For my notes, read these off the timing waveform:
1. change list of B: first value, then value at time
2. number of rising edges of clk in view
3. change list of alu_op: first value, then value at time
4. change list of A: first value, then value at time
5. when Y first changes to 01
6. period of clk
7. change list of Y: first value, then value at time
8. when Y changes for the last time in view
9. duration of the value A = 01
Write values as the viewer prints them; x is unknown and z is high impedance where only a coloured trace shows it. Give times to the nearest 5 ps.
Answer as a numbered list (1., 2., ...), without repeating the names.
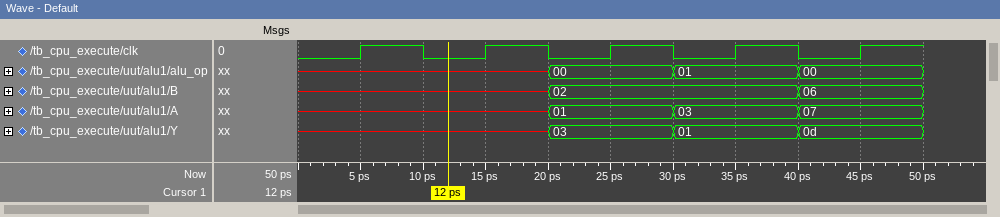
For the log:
1. x, 02 at 20 ps, 06 at 40 ps
2. 5
3. x, 00 at 20 ps, 01 at 30 ps, 00 at 40 ps
4. x, 01 at 20 ps, 03 at 30 ps, 07 at 40 ps
5. 30 ps
6. 10 ps
7. x, 03 at 20 ps, 01 at 30 ps, 0d at 40 ps
8. 40 ps
9. 10 ps
